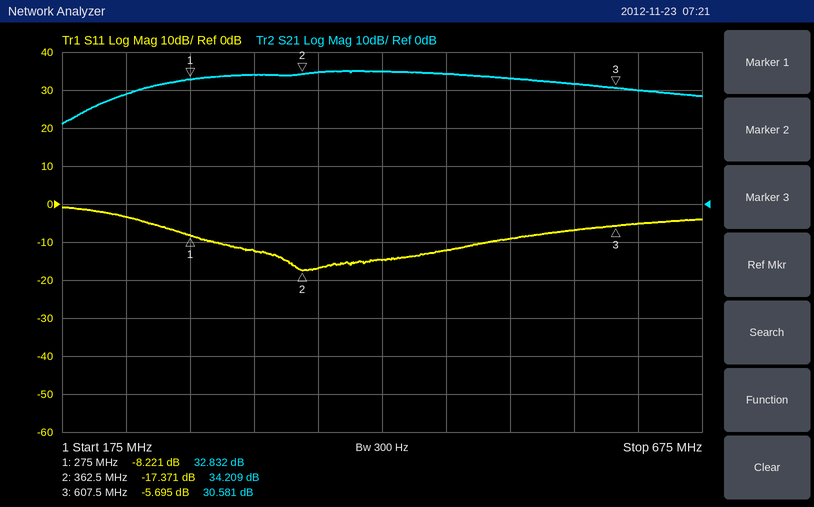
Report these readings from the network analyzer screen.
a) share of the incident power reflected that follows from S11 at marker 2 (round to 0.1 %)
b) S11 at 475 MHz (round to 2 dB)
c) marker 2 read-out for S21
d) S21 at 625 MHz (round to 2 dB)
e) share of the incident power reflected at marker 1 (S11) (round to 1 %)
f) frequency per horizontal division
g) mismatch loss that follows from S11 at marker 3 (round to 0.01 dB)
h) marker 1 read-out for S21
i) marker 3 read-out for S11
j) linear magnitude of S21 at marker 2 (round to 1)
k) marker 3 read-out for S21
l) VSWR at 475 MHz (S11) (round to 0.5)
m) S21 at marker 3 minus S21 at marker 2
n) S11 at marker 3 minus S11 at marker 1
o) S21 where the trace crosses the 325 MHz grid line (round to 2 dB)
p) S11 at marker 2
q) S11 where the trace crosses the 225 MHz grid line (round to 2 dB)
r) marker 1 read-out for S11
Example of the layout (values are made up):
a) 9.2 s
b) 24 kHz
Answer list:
a) 1.8 %
b) -12 dB
c) 34.209 dB
d) 30 dB
e) 15 %
f) 50 MHz
g) 1.36 dB
h) 32.832 dB
i) -5.695 dB
j) 51
k) 30.581 dB
l) 1.5
m) -3.628 dB
n) 2.526 dB
o) 34 dB
p) -17.371 dB
q) -4 dB
r) -8.221 dB
